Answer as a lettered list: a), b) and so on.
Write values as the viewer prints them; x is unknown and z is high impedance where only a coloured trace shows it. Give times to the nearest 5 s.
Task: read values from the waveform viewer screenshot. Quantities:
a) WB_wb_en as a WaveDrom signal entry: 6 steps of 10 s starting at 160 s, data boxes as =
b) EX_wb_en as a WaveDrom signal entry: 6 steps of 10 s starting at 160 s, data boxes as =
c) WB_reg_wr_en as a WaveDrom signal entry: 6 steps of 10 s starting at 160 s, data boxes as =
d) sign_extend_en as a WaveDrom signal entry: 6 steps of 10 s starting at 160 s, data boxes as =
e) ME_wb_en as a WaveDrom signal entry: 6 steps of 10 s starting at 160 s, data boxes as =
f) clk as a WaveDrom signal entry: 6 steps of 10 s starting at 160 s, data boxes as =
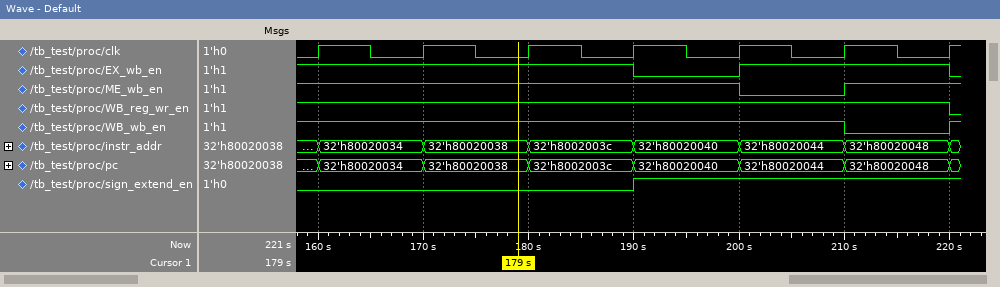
a) {name: 'WB_wb_en', wave: '1....0'}
b) {name: 'EX_wb_en', wave: '1..01.'}
c) {name: 'WB_reg_wr_en', wave: '1.....'}
d) {name: 'sign_extend_en', wave: '0..1..'}
e) {name: 'ME_wb_en', wave: '1...01'}
f) {name: 'clk', wave: 'p.....'}
